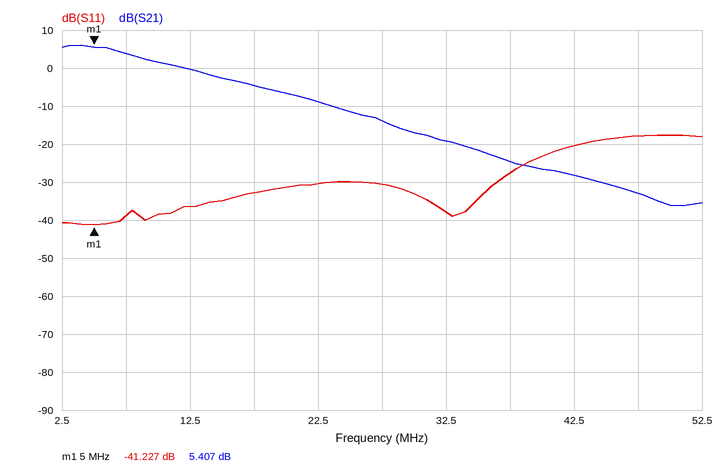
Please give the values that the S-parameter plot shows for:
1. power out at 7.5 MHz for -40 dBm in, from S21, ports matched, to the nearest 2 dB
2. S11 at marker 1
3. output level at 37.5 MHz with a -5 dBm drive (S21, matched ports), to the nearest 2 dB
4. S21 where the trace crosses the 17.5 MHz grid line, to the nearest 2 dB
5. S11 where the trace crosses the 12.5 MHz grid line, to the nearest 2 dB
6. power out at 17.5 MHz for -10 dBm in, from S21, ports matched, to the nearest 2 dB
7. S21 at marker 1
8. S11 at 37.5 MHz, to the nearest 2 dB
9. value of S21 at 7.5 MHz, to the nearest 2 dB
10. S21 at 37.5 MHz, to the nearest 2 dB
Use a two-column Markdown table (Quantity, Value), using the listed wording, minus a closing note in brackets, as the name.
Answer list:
| Quantity | Value |
|---|---|
| power out at 7.5 MHz for -40 dBm in, from S21, ports matched, to the nearest 2 dB | -36 dBm |
| S11 at marker 1 | -41.227 dB |
| output level at 37.5 MHz with a -5 dBm drive (S21, matched ports), to the nearest 2 dB | -30 dBm |
| S21 where the trace crosses the 17.5 MHz grid line, to the nearest 2 dB | -4 dB |
| S11 where the trace crosses the 12.5 MHz grid line, to the nearest 2 dB | -36 dB |
| power out at 17.5 MHz for -10 dBm in, from S21, ports matched, to the nearest 2 dB | -14 dBm |
| S21 at marker 1 | 5.407 dB |
| S11 at 37.5 MHz, to the nearest 2 dB | -28 dB |
| value of S21 at 7.5 MHz, to the nearest 2 dB | 4 dB |
| S21 at 37.5 MHz, to the nearest 2 dB | -24 dB |
